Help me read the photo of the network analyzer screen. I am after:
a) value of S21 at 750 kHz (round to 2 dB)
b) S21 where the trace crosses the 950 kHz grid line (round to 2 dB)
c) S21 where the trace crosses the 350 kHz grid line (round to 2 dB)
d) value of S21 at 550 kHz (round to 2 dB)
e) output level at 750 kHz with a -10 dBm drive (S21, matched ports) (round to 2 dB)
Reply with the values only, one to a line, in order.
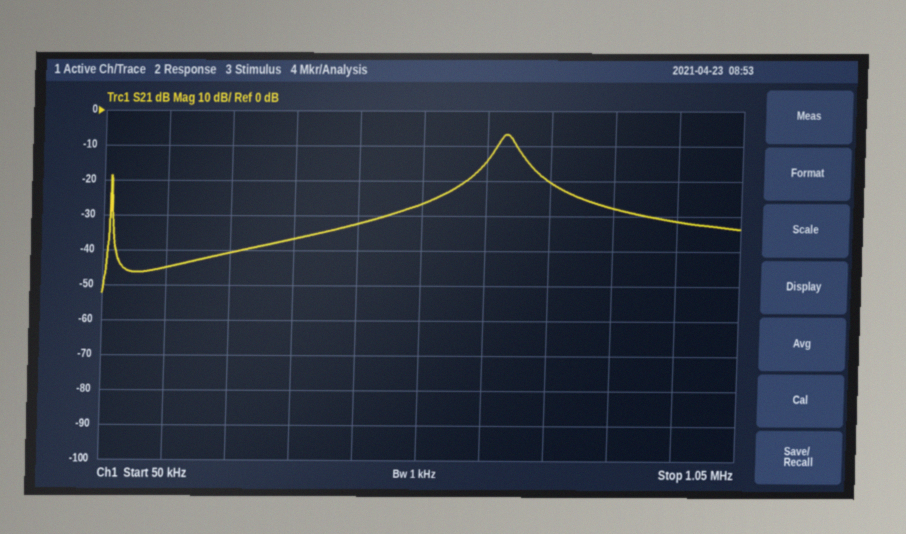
-20 dB
-32 dB
-36 dB
-26 dB
-30 dBm
